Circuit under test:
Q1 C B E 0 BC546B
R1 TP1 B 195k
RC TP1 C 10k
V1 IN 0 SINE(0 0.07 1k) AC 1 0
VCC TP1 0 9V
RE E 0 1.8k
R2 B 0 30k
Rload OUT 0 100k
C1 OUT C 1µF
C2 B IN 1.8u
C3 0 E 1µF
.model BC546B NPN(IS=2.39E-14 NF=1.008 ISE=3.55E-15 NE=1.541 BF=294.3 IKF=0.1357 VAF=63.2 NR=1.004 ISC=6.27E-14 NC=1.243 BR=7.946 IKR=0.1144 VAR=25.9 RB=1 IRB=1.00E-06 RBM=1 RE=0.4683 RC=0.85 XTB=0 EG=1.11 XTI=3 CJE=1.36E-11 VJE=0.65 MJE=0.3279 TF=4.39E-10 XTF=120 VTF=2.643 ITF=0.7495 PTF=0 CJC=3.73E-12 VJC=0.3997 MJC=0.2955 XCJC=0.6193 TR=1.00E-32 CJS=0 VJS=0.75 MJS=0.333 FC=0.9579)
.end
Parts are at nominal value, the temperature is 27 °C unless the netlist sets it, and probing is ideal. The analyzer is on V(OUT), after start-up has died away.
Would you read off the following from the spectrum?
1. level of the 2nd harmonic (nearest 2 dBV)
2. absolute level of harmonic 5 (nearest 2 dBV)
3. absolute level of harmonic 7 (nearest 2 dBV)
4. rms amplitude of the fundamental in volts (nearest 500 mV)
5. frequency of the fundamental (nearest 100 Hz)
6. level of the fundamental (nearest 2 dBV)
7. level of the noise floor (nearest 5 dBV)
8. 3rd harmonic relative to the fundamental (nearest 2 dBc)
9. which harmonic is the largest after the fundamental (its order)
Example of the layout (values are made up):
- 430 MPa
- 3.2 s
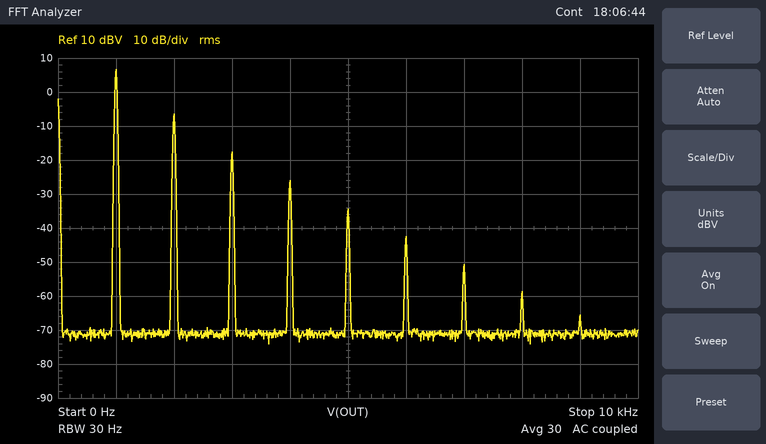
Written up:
- -6 dBV
- -34 dBV
- -50 dBV
- 2.0 V
- 1.0 kHz
- 6 dBV
- -70 dBV
- -24 dBc
- 2
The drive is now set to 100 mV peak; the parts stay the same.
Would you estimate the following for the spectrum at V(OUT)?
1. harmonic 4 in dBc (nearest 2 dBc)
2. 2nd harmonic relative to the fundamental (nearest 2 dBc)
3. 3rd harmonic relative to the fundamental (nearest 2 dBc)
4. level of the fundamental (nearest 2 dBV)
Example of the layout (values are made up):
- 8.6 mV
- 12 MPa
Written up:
- -26 dBc
- -10 dBc
- -20 dBc
- 8 dBV
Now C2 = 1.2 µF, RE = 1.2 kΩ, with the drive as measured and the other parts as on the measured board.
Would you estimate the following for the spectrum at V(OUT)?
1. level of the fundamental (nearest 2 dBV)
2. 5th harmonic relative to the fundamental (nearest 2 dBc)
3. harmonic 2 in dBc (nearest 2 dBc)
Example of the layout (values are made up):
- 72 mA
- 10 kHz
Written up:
- 8 dBV
- -48 dBc
- -18 dBc
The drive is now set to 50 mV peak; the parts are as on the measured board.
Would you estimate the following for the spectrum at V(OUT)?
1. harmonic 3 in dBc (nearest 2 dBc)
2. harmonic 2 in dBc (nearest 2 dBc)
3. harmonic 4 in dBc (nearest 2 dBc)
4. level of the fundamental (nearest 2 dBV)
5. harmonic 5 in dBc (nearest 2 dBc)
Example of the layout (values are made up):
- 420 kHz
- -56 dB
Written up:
- -30 dBc
- -16 dBc
- -40 dBc
- 4 dBV
- -52 dBc
